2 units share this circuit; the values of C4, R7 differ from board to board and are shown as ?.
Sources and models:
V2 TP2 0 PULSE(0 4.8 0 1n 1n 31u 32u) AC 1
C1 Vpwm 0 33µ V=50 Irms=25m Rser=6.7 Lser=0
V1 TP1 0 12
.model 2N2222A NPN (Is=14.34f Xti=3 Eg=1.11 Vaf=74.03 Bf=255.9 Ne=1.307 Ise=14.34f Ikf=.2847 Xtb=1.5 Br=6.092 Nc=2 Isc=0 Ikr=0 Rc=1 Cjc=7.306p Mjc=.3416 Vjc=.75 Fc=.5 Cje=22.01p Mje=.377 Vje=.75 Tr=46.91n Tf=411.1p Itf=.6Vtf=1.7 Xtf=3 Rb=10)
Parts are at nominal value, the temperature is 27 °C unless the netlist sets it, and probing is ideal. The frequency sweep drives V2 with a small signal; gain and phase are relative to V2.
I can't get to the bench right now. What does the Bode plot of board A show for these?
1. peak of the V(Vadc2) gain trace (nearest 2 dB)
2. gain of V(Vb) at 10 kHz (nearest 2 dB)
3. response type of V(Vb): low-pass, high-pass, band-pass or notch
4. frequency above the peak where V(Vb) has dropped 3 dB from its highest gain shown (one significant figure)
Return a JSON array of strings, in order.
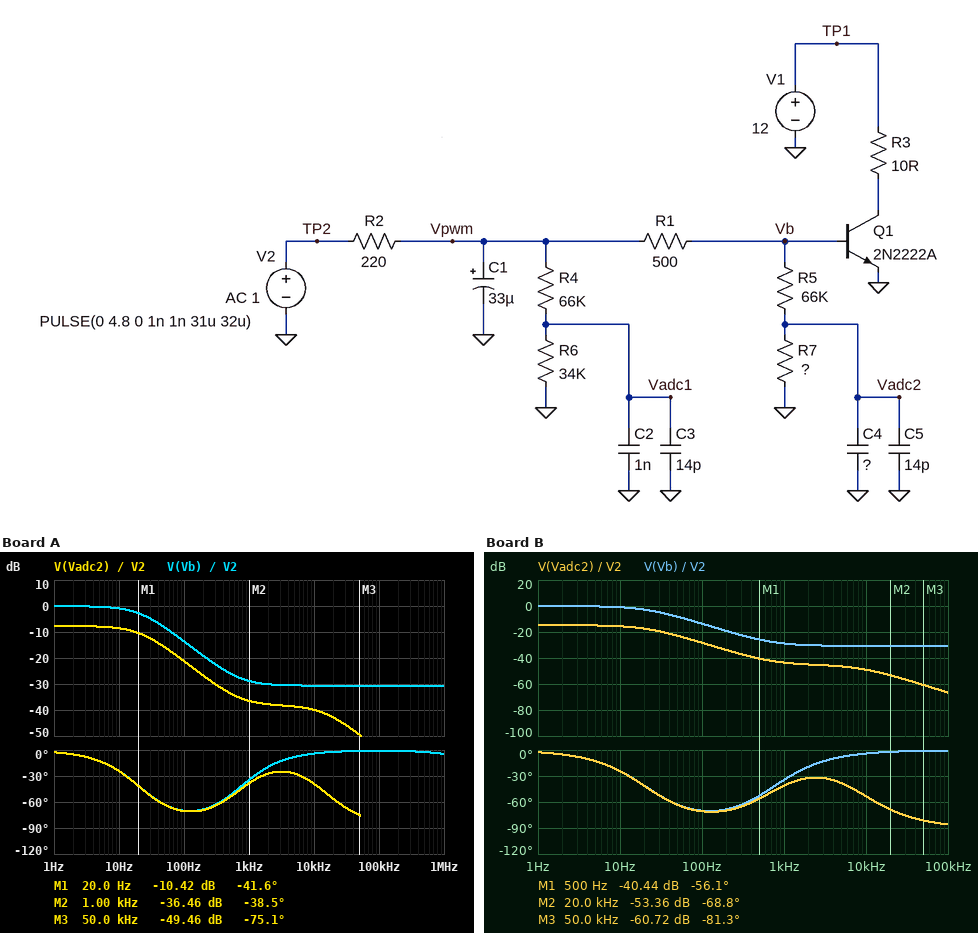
["-8 dB", "-30 dB", "low-pass", "20 Hz"]
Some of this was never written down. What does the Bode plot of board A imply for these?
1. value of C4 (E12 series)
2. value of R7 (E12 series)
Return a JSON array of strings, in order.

["390 pF", "47 kΩ"]
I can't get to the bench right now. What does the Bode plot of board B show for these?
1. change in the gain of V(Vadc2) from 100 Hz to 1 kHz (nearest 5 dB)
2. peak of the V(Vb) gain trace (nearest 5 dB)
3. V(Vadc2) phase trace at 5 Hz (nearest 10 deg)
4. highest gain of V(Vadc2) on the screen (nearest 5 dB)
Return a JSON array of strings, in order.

["-15 dB", "0 dB", "-10 deg", "-15 dB"]
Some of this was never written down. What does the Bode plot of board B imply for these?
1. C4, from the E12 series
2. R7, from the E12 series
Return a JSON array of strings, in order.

["1.5 nF", "15 kΩ"]
